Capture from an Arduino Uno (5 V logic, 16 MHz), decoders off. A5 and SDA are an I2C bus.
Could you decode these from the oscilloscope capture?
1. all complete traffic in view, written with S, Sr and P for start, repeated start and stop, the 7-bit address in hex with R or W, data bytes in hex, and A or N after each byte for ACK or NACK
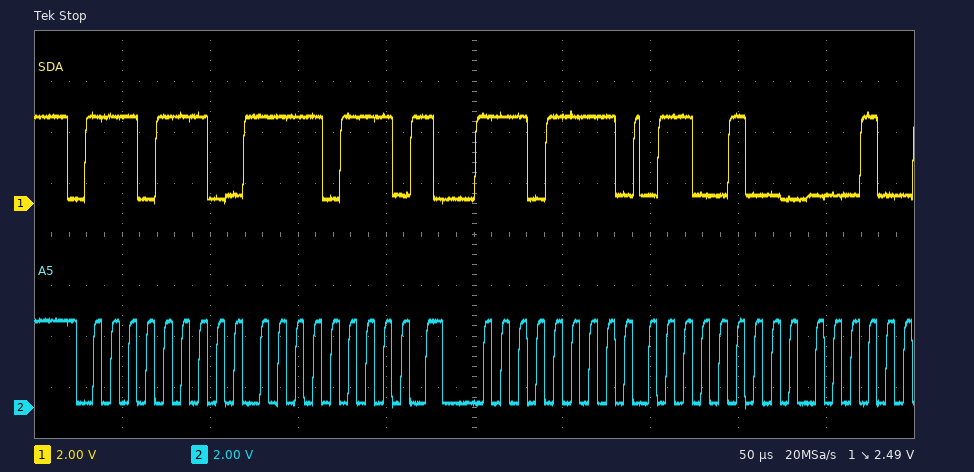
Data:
S 77W A F7 A Sr 77R A 64 A
